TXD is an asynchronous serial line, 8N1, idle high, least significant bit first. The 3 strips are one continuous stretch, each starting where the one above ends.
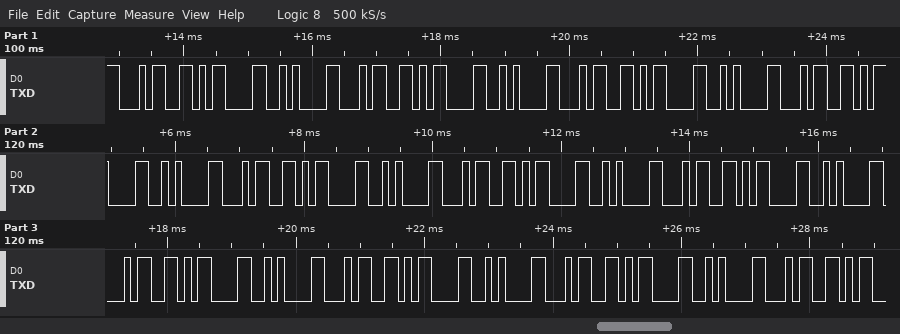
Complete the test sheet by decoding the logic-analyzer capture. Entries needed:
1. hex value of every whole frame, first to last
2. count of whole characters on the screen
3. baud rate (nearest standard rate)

0x34 0x0D 0x0A 0x34 0x0D 0x0A 0x34 0x0D 0x0A 0x34 0x0D 0x0A 0x34 0x0D 0x0A 0x34 0x0D 0x0A 0x34 0x0D 0x0A 0x34 0x0D 0x0A 0x34 0x0D 0x0A 0x34 0x0D 0x0A 0x34
31
9600 baud
